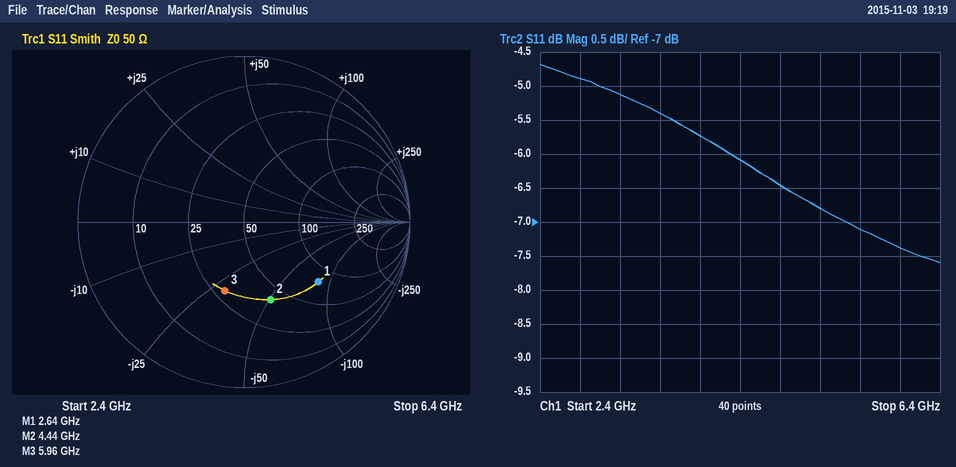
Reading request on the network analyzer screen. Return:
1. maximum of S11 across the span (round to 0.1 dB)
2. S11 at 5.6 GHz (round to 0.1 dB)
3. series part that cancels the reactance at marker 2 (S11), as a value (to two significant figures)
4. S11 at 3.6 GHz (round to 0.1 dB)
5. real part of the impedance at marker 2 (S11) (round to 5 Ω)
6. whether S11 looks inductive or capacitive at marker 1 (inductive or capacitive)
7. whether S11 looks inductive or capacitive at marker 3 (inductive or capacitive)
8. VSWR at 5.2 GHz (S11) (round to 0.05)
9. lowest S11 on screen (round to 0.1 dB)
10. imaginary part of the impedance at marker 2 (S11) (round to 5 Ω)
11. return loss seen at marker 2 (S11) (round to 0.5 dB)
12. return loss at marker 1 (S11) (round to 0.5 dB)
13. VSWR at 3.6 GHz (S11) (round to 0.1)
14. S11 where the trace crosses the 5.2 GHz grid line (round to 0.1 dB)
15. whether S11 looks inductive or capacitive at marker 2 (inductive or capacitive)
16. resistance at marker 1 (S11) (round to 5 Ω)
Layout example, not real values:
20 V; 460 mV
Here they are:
-4.7 dB; -7.1 dB; 1.8 nH; -5.4 dB; 40 Ω; capacitive; capacitive; 2.70; -7.6 dB; -50 Ω; 6.0 dB; 5.0 dB; 3.3; -6.8 dB; capacitive; 75 Ω
